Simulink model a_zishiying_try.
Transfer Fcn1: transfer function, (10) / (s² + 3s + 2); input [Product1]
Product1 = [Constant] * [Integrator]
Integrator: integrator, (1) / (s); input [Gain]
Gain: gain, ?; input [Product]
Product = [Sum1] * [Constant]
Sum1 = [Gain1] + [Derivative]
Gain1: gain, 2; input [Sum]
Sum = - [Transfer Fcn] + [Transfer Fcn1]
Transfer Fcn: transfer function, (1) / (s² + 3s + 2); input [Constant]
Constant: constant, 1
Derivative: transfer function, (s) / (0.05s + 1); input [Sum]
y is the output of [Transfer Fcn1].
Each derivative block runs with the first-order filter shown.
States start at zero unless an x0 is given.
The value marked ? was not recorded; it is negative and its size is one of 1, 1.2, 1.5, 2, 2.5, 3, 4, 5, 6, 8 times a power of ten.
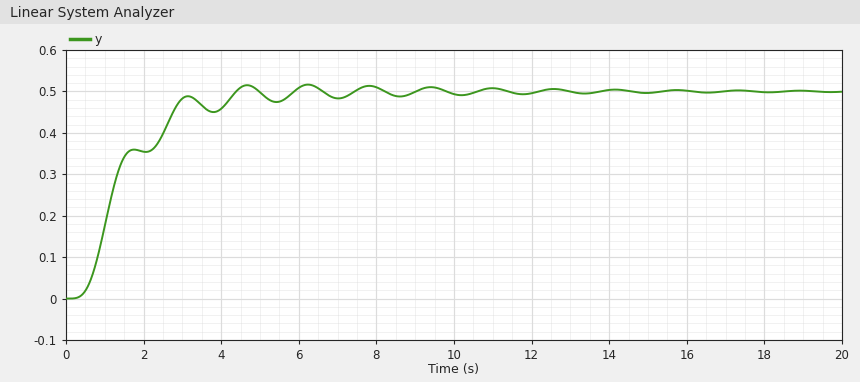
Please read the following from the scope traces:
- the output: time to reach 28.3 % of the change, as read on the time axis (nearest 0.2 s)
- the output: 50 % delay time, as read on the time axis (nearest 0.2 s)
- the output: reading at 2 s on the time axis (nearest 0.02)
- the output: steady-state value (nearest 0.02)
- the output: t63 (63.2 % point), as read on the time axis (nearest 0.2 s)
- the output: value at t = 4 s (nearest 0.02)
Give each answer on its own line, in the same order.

1.0 s
1.2 s
0.36
0.50
1.4 s
0.46
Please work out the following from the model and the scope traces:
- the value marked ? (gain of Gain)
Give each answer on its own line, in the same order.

-1.5
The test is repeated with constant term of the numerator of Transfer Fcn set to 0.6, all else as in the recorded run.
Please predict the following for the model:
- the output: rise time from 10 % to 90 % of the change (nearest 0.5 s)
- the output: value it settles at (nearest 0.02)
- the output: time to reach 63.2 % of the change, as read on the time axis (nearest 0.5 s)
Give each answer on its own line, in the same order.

2.0 s
0.30
1.5 s
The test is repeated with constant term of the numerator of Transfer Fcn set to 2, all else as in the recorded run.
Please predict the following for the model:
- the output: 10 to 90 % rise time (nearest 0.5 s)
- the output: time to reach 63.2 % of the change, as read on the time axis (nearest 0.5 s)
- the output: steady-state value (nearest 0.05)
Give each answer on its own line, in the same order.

2.0 s
1.5 s
1.00
